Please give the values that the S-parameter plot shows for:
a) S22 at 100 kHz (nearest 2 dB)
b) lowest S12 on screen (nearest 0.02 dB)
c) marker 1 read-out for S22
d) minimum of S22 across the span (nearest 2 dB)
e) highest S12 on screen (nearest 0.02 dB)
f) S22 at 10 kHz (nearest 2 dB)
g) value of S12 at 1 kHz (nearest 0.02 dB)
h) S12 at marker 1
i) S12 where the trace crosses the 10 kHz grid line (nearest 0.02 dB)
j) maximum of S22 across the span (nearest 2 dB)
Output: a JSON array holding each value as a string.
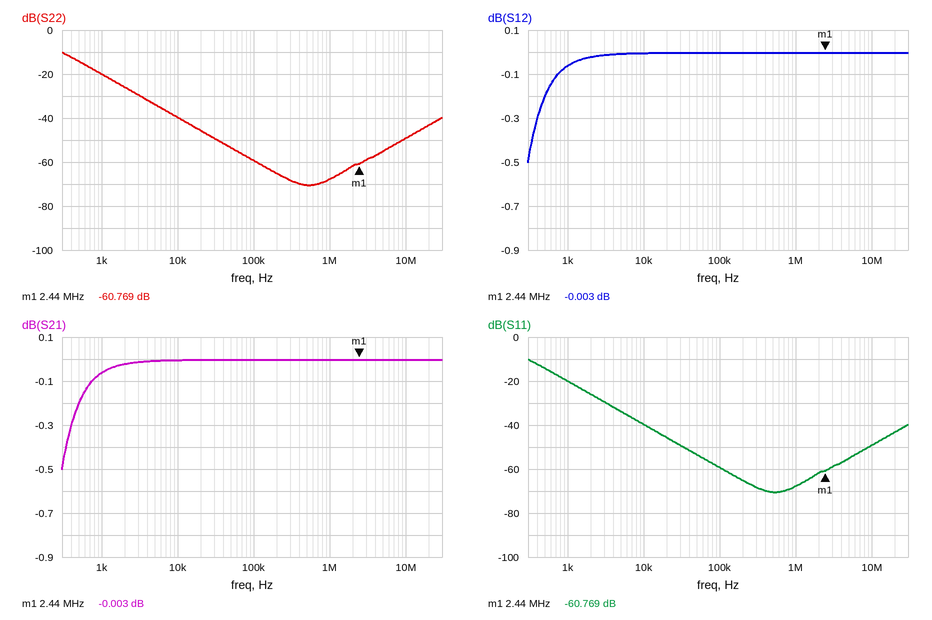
["-60 dB", "-0.50 dB", "-60.769 dB", "-70 dB", "0.00 dB", "-40 dB", "-0.06 dB", "-0.003 dB", "0.00 dB", "-10 dB"]
